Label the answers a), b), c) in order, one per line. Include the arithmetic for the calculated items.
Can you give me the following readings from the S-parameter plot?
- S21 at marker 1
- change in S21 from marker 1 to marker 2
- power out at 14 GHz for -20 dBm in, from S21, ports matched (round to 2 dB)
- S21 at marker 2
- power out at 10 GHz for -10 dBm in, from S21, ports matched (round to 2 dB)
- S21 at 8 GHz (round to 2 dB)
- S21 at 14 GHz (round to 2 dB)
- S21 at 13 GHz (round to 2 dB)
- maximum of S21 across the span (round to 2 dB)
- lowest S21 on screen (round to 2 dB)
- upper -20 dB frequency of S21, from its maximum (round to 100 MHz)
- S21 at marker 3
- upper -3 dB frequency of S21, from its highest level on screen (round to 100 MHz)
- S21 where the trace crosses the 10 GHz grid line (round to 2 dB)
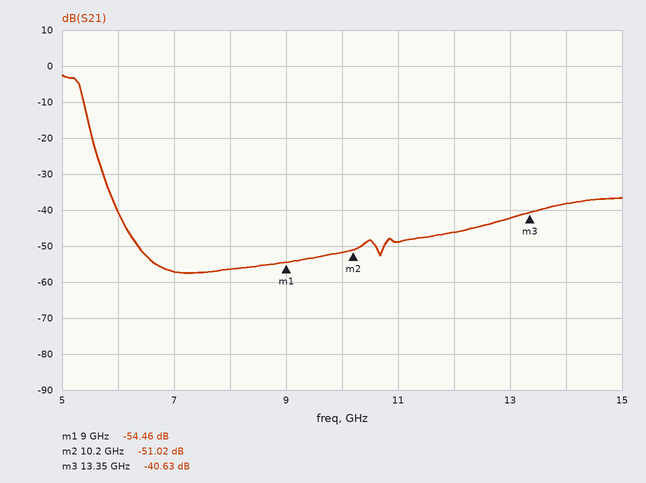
a) -54.46 dB
b) -51.02 − (-54.46) = 3.44 dB
c) -20 dBm + (-38 dB) = -58 dBm
d) -51.02 dB
e) -10 dBm + (-52 dB) = -62 dBm
f) -56 dB
g) -38 dB
h) -42 dB
i) -2 dB
j) -58 dB
k) 5.6 GHz
l) -40.63 dB
m) 5.3 GHz
n) -52 dB
